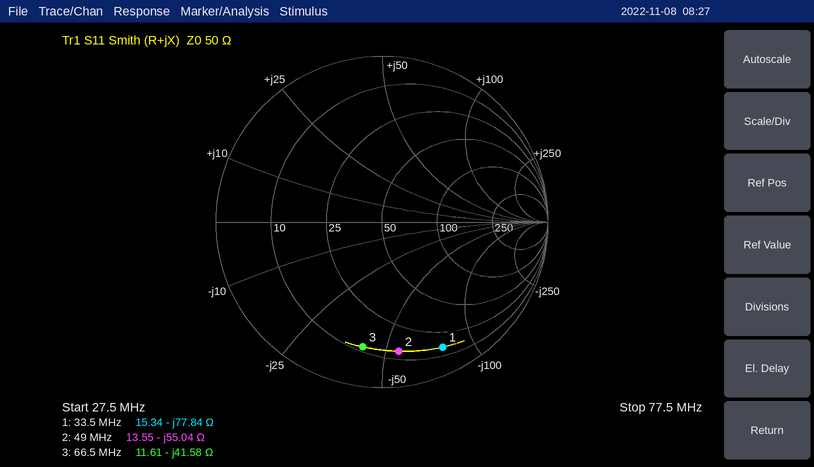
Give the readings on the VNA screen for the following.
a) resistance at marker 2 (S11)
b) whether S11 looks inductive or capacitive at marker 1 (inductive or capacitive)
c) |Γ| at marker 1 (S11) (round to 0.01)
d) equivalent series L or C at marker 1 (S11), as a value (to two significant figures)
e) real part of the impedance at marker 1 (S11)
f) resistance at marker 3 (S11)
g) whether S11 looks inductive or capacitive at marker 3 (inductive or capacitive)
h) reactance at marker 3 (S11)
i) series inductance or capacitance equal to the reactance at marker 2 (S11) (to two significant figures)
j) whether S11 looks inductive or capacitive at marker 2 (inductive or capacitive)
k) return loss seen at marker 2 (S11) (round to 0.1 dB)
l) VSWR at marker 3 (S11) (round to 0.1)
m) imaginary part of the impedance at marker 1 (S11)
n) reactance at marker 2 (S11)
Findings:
13.55 Ω
capacitive
0.84
61 pF
15.34 Ω
11.61 Ω
capacitive
-41.58 Ω
59 pF
capacitive
2.1 dB
7.4
-77.84 Ω
-55.04 Ω
